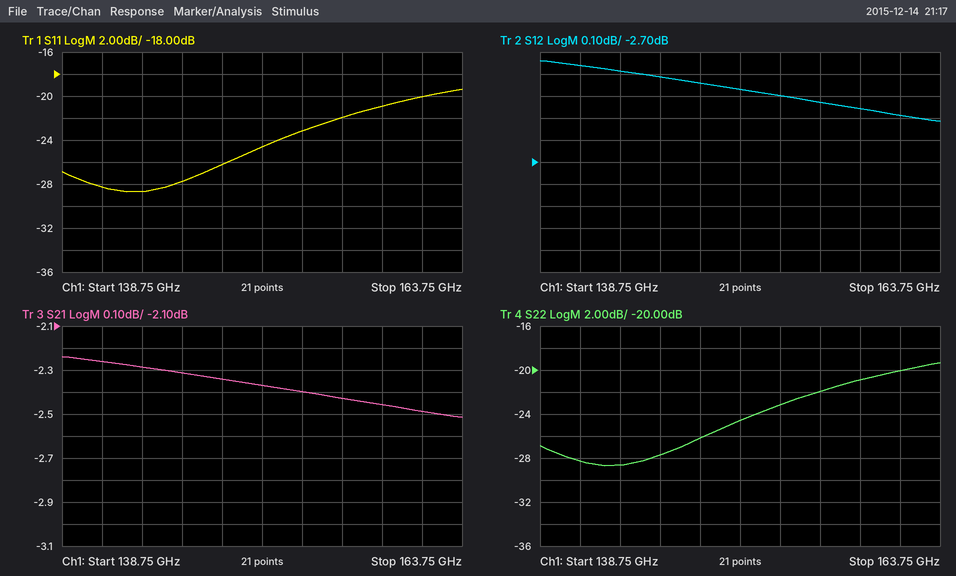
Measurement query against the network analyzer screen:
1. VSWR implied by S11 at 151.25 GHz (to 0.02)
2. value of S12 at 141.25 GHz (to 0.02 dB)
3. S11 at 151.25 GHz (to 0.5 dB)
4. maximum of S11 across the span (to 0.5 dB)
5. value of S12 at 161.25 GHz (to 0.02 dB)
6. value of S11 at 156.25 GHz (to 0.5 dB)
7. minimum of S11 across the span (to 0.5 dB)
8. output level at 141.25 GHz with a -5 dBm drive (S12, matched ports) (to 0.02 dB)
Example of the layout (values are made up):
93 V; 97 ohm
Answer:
1.12; -2.26 dB; -24.5 dB; -19.5 dB; -2.48 dB; -22.0 dB; -28.5 dB; -7.26 dBm
